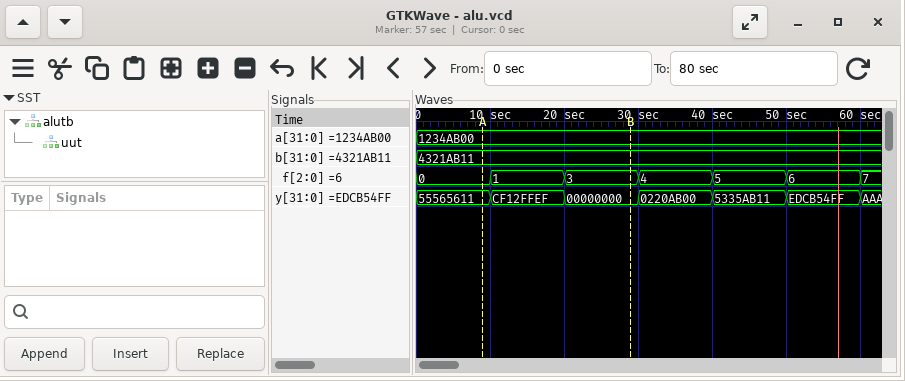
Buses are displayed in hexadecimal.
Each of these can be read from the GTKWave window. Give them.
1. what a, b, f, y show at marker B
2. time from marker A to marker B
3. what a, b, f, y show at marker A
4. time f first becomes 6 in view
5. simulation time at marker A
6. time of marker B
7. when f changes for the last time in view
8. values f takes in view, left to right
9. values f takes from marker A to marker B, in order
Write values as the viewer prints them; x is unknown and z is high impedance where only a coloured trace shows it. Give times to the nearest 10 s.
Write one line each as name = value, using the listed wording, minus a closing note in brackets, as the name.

what a, b, f, y show at marker B = a=1234AB00, b=4321AB11, f=3, y=00000000
time from marker A to marker B = 20 s
what a, b, f, y show at marker A = a=1234AB00, b=4321AB11, f=0, y=55565611
time f first becomes 6 in view = 50 s
simulation time at marker A = 10 s
time of marker B = 30 s
when f changes for the last time in view = 60 s
values f takes in view, left to right = 0, 1, 3, 4, 5, 6, 7
values f takes from marker A to marker B, in order = 0, 1, 3
